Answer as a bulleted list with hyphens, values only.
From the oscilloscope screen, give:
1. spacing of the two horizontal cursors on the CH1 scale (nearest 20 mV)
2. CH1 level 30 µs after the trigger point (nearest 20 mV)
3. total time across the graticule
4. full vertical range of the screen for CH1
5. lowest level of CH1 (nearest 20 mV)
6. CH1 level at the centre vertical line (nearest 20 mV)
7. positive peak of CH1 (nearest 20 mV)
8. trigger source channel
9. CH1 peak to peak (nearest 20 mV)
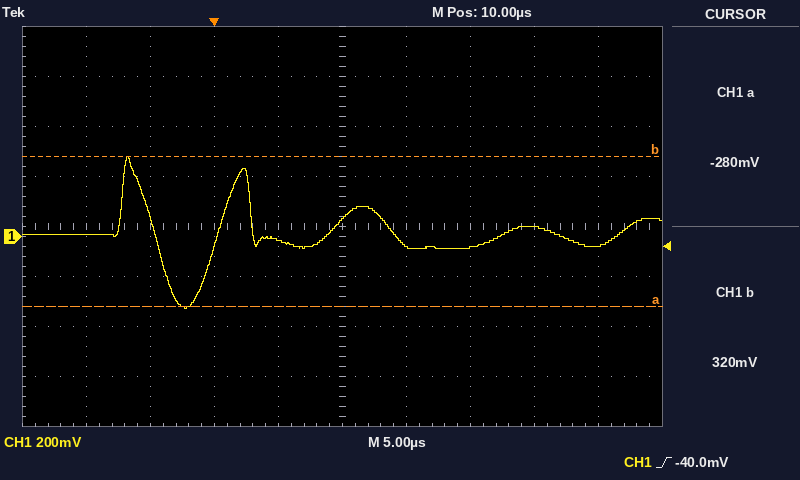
- 600 mV
- -40 mV
- 50 µs
- 1.6 V
- -280 mV
- 60 mV
- 320 mV
- CH1
- 600 mV
